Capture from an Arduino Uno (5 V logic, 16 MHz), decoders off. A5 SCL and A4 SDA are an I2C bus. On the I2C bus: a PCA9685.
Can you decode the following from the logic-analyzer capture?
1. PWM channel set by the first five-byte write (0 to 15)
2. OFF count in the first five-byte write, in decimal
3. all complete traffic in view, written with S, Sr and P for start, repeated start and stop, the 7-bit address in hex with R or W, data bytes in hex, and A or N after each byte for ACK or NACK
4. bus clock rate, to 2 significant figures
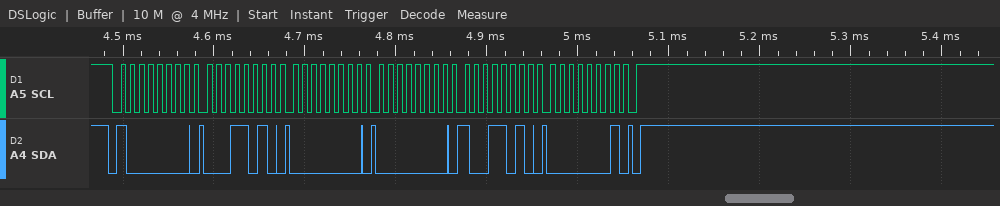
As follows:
5
410
S 40W A 1A A 00 A 00 A 9A A 01 A P
100 kHz
